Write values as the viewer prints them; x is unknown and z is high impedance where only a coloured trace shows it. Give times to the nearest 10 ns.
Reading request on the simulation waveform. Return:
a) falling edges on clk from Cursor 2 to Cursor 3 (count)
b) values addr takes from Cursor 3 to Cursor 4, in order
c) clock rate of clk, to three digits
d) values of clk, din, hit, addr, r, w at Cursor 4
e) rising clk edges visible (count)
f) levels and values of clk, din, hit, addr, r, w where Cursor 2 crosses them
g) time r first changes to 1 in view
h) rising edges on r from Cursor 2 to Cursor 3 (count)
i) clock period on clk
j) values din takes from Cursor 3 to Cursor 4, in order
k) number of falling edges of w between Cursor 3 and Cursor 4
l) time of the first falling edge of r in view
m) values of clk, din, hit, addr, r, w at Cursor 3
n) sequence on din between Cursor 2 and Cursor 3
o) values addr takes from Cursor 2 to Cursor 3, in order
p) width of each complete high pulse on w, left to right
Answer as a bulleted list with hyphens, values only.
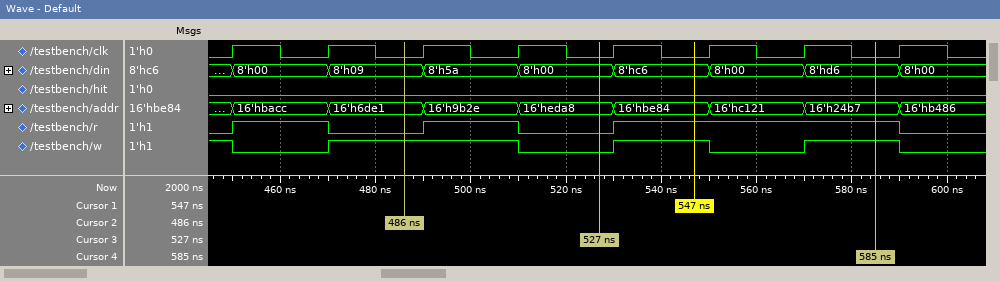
- 2
- 16'heda8, 16'hbe84, 16'hc121, 16'h24b7
- 50.0 MHz
- clk=0, din=8'hd6, hit=0, addr=16'h24b7, r=1, w=1
- 8
- clk=0, din=8'h09, hit=0, addr=16'h6de1, r=0, w=1
- 450 ns
- 1
- 20 ns
- 8'h00, 8'hc6, 8'h00, 8'hd6
- 1
- 470 ns
- clk=0, din=8'h00, hit=0, addr=16'heda8, r=0, w=0
- 8'h09, 8'h5a, 8'h00
- 16'h6de1, 16'h9b2e, 16'heda8
- 40 ns, 20 ns, 20 ns
